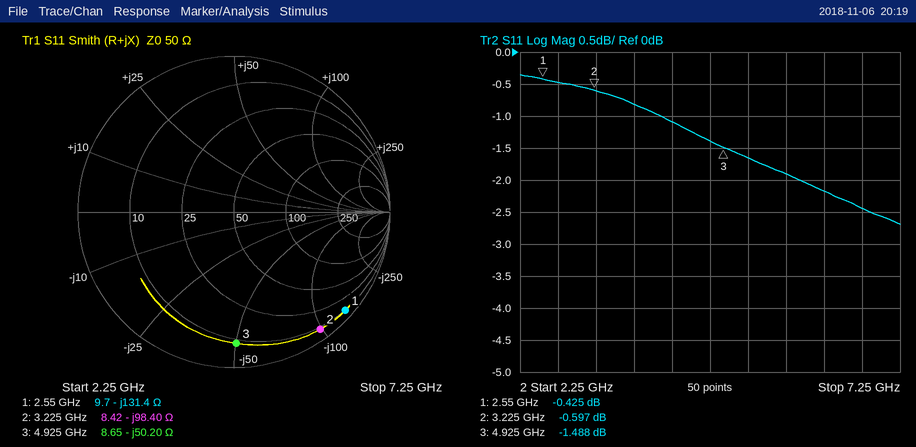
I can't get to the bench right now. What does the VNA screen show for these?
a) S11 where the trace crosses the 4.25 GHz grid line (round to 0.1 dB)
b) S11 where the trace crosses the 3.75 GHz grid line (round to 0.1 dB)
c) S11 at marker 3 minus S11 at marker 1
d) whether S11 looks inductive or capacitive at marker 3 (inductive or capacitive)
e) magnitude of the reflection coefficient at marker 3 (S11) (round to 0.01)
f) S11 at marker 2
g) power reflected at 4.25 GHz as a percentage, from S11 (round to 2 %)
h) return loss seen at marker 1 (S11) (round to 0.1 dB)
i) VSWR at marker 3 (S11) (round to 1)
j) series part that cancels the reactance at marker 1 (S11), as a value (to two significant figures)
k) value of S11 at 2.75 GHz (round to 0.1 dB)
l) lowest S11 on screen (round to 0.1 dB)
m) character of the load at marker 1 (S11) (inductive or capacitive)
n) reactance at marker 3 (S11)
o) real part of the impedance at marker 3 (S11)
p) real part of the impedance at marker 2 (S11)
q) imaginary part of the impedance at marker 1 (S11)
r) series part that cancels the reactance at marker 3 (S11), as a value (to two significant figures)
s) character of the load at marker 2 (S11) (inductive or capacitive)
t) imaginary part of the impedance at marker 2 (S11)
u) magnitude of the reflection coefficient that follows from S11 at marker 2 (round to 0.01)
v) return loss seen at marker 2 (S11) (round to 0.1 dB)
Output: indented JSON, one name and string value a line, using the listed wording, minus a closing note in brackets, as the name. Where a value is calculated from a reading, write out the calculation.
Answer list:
{
  "S11 where the trace crosses the 4.25 GHz grid line": "-1.1 dB",
  "S11 where the trace crosses the 3.75 GHz grid line": "-0.8 dB",
  "S11 at marker 3 minus S11 at marker 1": "-1.488 − (-0.425) = -1.063 dB",
  "whether S11 looks inductive or capacitive at marker 3": "capacitive",
  "magnitude of the reflection coefficient at marker 3 (S11)": "0.84",
  "S11 at marker 2": "-0.597 dB",
  "power reflected at 4.25 GHz as a percentage, from S11": "10^(-1.1/10) ≈ 78 %",
  "return loss seen at marker 1 (S11)": "0.4 dB",
  "VSWR at marker 3 (S11)": "(1 + 0.8426)/(1 − 0.8426) ≈ 12",
  "series part that cancels the reactance at marker 1 (S11), as a value": "L = 131.4 Ω/(2π × 2.55 GHz) ≈ 8.2 nH",
  "value of S11 at 2.75 GHz": "-0.5 dB",
  "lowest S11 on screen": "-2.7 dB",
  "character of the load at marker 1 (S11)": "capacitive",
  "reactance at marker 3": "-50.20 Ω",
  "real part of the impedance at marker 3": "8.65 Ω",
  "real part of the impedance at marker 2": "8.42 Ω",
  "imaginary part of the impedance at marker 1": "-131.4 Ω",
  "series part that cancels the reactance at marker 3 (S11), as a value": "L = 50.2 Ω/(2π × 4.925 GHz) ≈ 1.6 nH",
  "character of the load at marker 2 (S11)": "capacitive",
  "imaginary part of the impedance at marker 2": "-98.40 Ω",
  "magnitude of the reflection coefficient that follows from S11 at marker 2": "10^(-0.597/20) ≈ 0.93",
  "return loss seen at marker 2 (S11)": "0.6 dB"
}
